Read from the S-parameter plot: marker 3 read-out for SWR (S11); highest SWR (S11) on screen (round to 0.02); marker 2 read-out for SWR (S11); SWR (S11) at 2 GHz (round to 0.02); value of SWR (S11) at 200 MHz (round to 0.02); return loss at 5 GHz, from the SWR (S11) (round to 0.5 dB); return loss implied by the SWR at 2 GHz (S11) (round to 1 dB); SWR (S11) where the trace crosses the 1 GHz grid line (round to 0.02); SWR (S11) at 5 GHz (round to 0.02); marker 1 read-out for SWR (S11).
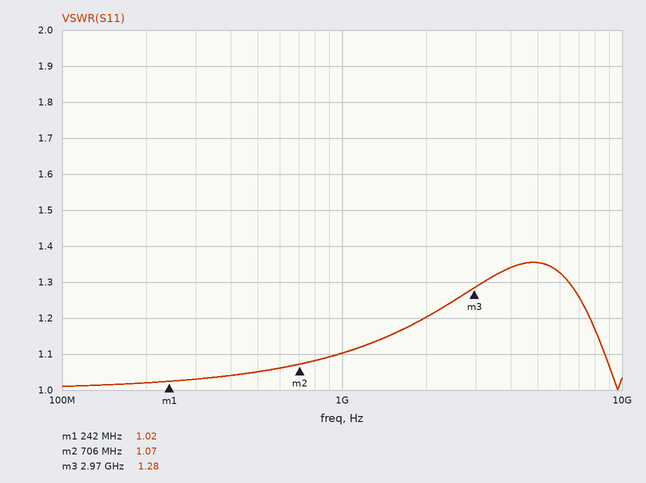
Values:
1.28
1.36
1.07
1.20
1.02
16.5 dB
21 dB
1.10
1.36
1.02
